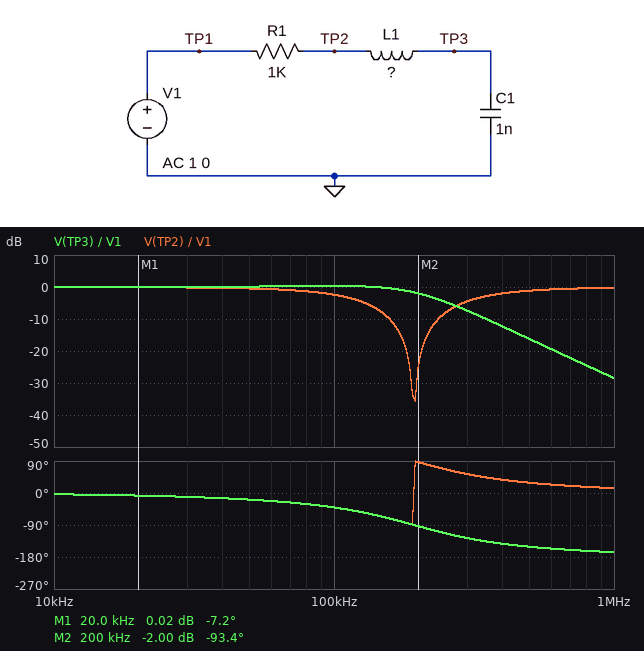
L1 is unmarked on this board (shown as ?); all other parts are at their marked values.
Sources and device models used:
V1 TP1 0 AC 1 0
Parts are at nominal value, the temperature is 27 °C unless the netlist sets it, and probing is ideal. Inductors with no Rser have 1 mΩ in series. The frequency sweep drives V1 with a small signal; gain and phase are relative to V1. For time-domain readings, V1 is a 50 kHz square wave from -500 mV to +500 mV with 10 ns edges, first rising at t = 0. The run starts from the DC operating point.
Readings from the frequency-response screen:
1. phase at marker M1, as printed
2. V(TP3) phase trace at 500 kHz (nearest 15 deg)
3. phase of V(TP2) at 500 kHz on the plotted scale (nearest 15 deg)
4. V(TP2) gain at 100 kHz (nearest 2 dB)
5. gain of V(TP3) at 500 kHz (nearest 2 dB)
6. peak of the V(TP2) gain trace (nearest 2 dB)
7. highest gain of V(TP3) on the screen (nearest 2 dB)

-7.2 deg
-150 deg
30 deg
-2 dB
-16 dB
0 dB
0 dB
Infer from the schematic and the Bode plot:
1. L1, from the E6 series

680 µH
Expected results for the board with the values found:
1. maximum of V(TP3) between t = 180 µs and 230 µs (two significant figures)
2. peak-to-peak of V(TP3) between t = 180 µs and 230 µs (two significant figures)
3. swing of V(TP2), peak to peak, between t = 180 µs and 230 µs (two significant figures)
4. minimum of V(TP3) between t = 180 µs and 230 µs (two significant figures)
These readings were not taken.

590 mV
1.2 V
1.1 V
-590 mV
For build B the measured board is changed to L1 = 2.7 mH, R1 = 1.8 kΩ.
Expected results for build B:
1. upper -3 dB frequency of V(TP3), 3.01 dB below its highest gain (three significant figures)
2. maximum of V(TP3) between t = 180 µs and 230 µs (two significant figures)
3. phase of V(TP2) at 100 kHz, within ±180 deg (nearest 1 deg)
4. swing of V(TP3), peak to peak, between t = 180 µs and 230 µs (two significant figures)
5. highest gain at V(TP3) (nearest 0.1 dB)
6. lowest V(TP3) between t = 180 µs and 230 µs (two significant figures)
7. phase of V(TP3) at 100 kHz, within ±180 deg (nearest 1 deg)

111 kHz
630 mV
87 deg
1.3 V
0.8 dB
-630 mV
-93 deg
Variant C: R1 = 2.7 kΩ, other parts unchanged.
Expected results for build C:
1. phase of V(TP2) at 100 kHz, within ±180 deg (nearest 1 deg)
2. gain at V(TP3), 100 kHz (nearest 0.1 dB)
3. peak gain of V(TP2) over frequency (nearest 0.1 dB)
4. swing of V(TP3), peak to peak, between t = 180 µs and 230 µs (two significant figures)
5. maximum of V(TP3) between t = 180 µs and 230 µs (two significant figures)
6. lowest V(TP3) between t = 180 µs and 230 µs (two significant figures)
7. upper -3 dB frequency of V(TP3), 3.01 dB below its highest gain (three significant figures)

-67 deg
-5.3 dB
0 dB
960 mV
480 mV
-480 mV
64.9 kHz
